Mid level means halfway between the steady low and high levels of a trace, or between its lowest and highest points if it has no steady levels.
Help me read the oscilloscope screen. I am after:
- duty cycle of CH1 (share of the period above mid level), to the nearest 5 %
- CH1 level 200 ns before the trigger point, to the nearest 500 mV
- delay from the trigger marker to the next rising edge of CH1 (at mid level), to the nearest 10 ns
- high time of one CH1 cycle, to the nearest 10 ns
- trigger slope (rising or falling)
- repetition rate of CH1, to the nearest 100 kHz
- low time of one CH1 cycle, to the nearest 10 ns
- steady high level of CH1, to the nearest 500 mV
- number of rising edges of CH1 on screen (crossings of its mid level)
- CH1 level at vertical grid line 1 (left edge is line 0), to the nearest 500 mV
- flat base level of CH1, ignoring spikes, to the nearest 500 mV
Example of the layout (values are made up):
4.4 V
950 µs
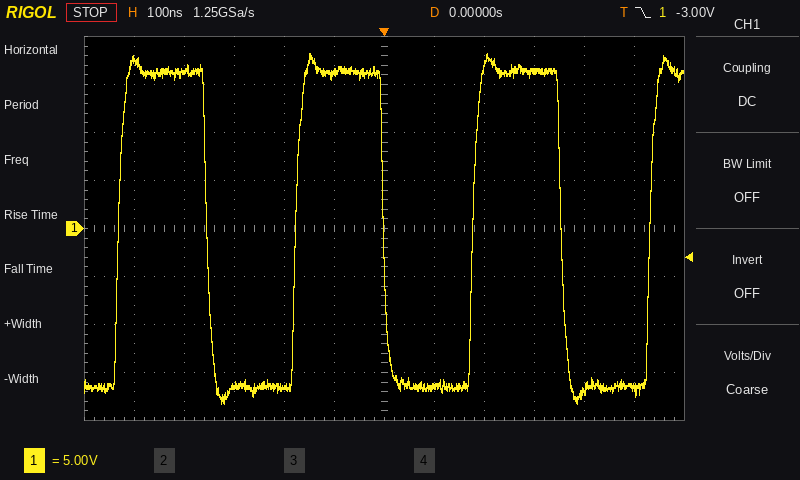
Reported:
50 %
-16.5 V
180 ns
180 ns
falling
2.8 MHz
180 ns
16.5 V
4
17.5 V
-16.5 V
